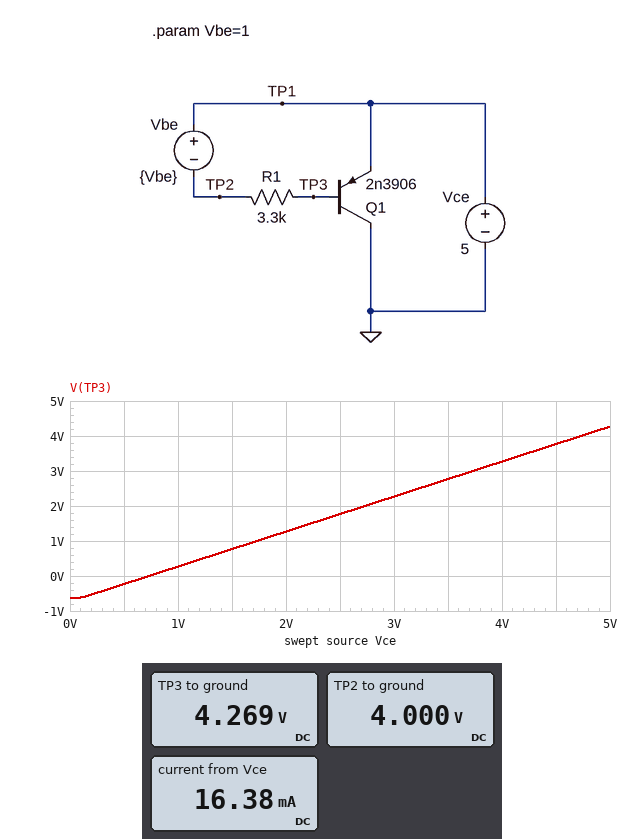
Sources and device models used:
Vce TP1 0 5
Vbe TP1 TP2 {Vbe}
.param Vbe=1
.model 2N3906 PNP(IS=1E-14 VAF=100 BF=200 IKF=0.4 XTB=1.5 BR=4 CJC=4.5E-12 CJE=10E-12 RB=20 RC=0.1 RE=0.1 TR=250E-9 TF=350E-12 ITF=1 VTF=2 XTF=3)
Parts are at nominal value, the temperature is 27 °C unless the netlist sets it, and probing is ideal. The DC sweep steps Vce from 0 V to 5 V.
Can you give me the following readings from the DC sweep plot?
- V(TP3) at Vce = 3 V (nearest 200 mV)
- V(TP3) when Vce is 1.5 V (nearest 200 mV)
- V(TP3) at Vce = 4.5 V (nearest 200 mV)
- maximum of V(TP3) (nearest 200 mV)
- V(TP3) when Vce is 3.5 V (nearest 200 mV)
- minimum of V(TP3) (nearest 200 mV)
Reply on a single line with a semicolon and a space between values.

2.2 V; 800 mV; 3.8 V; 4.2 V; 2.8 V; -600 mV
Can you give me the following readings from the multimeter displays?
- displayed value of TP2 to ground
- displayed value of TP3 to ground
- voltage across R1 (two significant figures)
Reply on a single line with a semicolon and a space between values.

4.000 V; 4.269 V; 270 mV
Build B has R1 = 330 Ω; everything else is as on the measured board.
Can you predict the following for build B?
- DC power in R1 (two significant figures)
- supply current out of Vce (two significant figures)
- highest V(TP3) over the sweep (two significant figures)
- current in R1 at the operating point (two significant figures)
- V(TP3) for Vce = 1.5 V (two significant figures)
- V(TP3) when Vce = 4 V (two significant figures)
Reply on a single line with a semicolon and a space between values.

120 µW; 100 mA; 4.2 V; 600 µA; 700 mV; 3.2 V
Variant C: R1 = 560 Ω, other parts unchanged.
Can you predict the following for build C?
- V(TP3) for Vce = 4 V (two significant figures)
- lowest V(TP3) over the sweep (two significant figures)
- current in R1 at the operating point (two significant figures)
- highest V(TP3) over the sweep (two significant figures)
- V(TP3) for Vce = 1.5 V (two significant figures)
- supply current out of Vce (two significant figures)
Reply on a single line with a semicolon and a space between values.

3.2 V; -690 mV; 390 µA; 4.2 V; 720 mV; 69 mA
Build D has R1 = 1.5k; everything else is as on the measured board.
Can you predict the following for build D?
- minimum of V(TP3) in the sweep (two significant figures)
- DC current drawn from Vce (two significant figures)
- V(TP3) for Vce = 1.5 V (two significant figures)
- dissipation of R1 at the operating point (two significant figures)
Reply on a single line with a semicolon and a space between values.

-660 mV; 32 mA; 750 mV; 41 µW
